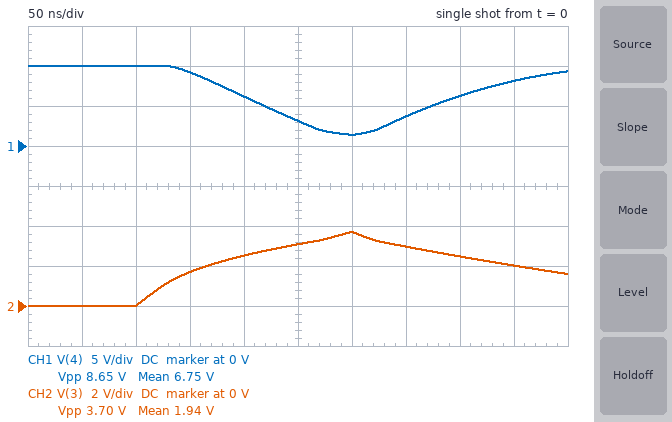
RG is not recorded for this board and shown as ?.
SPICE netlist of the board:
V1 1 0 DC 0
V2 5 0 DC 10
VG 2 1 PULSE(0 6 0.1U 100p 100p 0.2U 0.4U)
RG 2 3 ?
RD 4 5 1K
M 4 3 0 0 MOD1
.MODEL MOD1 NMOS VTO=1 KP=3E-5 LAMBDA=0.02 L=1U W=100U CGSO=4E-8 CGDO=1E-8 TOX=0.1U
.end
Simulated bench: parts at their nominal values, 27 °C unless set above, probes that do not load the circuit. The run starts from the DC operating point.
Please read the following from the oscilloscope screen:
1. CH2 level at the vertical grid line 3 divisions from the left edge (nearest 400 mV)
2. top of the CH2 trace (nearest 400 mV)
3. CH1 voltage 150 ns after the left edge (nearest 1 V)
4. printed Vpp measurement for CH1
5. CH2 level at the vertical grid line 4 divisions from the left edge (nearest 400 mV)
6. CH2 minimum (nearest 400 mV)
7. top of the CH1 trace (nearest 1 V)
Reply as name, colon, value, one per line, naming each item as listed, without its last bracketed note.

CH2 level at the vertical grid line 3 divisions from the left edge: 1.6 V
top of the CH2 trace: 3.6 V
CH1 voltage 150 ns after the left edge: 9 V
printed Vpp measurement for CH1: 8.65 V
CH2 level at the vertical grid line 4 divisions from the left edge: 2.4 V
CH2 minimum: 0 V
top of the CH1 trace: 10 V
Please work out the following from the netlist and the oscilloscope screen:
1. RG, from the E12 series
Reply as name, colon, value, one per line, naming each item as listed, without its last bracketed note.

RG, from the E12 series: 27 kΩ
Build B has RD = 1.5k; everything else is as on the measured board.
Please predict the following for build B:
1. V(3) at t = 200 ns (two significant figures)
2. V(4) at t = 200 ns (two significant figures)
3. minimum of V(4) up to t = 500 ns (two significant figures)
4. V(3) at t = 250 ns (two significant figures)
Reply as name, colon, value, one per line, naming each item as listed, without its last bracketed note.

V(3) at t = 200 ns: 2.4 V
V(4) at t = 200 ns: 5.3 V
minimum of V(4) up to t = 500 ns: 870 mV
V(3) at t = 250 ns: 2.9 V
